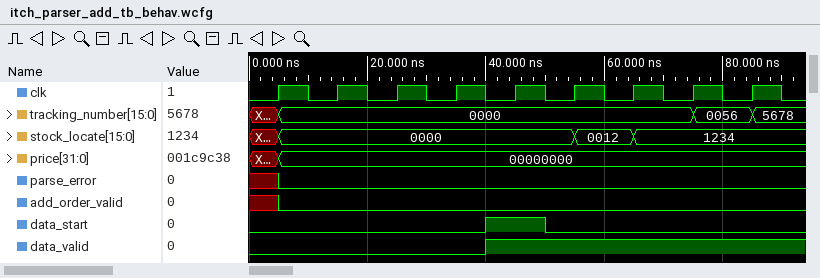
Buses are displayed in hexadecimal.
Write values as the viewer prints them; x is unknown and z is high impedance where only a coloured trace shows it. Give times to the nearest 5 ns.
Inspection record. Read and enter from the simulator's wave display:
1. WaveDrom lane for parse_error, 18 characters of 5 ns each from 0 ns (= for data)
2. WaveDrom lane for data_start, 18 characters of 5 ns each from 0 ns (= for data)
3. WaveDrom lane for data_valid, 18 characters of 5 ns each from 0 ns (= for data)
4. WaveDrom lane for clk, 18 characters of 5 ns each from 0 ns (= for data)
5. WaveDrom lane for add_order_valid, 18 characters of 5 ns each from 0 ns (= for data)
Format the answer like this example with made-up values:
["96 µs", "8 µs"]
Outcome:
["{name: 'parse_error', wave: 'x0................'}", "{name: 'data_start', wave: '0.......1.0.......'}", "{name: 'data_valid', wave: '0.......1.........'}", "{name: 'clk', wave: '010101010101010101'}", "{name: 'add_order_valid', wave: 'x0................'}"]
